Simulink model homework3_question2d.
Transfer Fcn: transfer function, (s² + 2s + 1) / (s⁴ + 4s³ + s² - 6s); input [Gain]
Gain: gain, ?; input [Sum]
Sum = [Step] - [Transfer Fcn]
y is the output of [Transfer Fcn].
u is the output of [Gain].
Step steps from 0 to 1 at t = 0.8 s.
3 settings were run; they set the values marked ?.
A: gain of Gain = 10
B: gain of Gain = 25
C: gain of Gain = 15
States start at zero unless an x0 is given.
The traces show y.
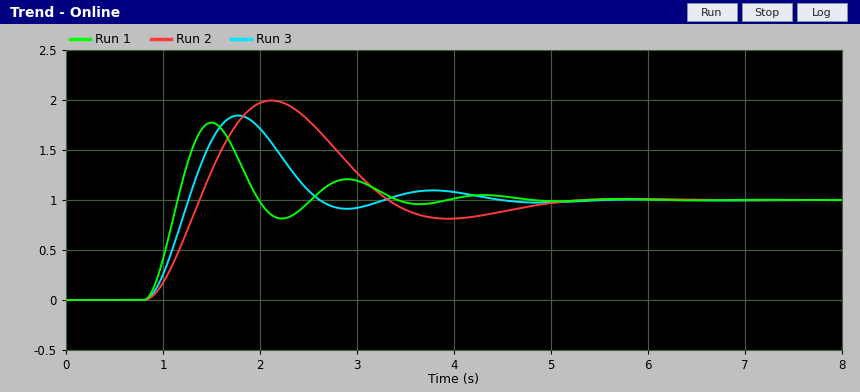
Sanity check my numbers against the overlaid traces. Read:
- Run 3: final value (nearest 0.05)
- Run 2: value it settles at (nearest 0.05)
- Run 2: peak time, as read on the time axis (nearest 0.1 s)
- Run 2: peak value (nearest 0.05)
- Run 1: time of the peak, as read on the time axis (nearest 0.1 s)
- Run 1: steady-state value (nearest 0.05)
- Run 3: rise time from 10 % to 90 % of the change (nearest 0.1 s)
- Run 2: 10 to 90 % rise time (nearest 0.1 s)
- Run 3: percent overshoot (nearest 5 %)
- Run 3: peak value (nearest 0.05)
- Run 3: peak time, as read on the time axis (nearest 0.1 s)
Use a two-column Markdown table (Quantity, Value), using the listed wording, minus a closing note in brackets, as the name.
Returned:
| Quantity | Value |
|---|---|
| Run 3: final value | 1.00 |
| Run 2: value it settles at | 1.00 |
| Run 2: peak time, as read on the time axis | 2.1 s |
| Run 2: peak value | 2.00 |
| Run 1: time of the peak, as read on the time axis | 1.5 s |
| Run 1: steady-state value | 1.00 |
| Run 3: rise time from 10 % to 90 % of the change | 0.3 s |
| Run 2: 10 to 90 % rise time | 0.4 s |
| Run 3: percent overshoot | 85 % |
| Run 3: peak value | 1.85 |
| Run 3: peak time, as read on the time axis | 1.8 s |
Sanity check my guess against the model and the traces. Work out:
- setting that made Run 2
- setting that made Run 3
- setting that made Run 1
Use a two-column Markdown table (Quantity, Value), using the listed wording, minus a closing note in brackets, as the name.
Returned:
| Quantity | Value |
|---|---|
| setting that made Run 2 | A |
| setting that made Run 3 | C |
| setting that made Run 1 | B |
